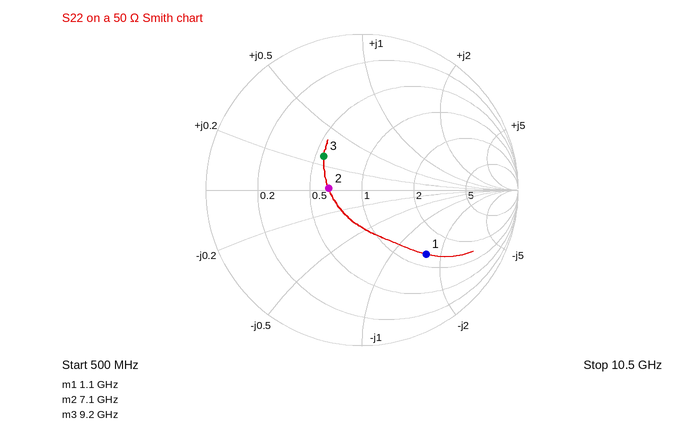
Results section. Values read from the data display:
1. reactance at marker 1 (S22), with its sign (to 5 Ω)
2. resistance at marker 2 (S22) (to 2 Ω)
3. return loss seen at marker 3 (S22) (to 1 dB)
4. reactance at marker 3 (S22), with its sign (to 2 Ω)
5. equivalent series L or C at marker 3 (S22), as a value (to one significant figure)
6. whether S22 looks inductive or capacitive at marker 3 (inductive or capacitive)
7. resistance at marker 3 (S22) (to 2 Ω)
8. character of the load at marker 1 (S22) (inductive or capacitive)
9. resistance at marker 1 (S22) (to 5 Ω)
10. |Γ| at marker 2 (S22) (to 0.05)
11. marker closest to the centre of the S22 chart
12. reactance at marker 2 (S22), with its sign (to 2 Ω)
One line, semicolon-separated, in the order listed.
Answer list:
-80 Ω; 32 Ω; 10 dB; +14 Ω; 200 pH; inductive; 28 Ω; capacitive; 65 Ω; 0.20; marker 2; 0 Ω
